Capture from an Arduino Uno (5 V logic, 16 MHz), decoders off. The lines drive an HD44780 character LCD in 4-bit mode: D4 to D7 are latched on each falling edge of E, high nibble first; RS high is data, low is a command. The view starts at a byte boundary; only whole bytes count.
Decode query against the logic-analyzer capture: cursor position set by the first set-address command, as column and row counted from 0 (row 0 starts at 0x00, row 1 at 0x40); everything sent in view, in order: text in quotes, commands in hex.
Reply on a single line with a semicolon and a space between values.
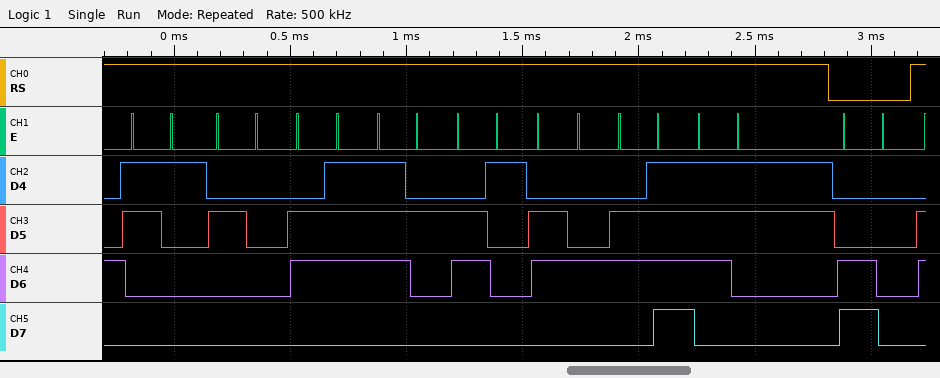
column 0, row 1; "1 grados" 0xC0
